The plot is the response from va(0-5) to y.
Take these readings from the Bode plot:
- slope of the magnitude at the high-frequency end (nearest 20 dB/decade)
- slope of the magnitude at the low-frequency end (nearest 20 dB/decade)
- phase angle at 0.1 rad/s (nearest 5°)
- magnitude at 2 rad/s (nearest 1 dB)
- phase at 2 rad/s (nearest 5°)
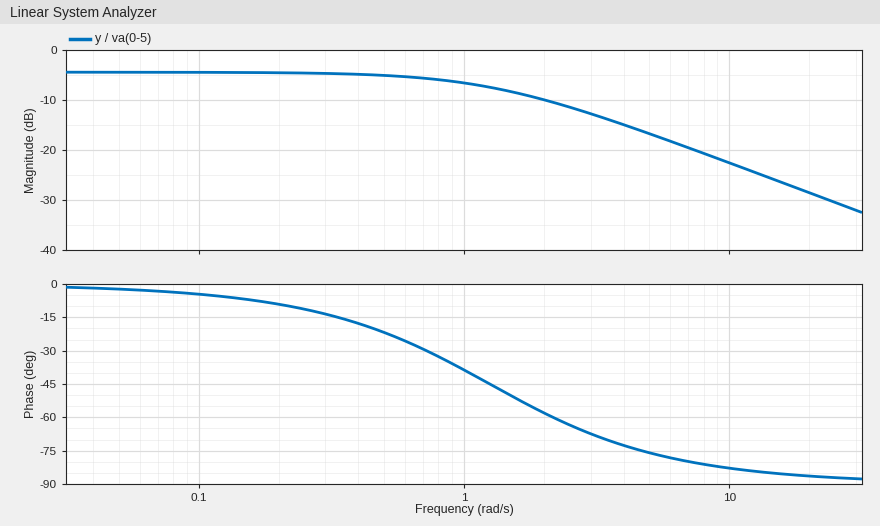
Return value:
-20 dB/decade
0 dB/decade
-5°
-10 dB
-60°
